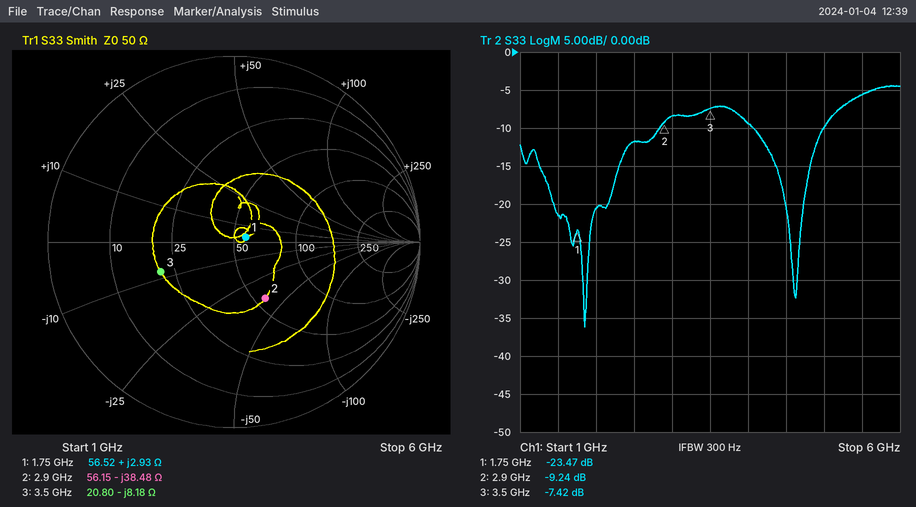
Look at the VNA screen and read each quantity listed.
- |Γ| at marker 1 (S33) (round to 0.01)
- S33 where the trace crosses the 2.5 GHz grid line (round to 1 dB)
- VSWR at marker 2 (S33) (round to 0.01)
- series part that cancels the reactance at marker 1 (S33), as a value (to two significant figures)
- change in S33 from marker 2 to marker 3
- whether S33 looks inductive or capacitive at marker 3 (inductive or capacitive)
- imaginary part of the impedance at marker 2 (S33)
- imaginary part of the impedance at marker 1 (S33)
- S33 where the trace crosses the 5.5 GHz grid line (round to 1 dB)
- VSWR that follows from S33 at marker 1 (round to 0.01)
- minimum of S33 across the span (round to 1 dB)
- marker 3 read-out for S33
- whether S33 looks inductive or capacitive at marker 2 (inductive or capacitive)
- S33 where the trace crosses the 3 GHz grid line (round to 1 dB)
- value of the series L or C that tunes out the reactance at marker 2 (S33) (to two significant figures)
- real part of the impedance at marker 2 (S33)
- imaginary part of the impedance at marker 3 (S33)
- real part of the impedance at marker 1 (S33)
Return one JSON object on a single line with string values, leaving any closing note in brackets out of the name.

{"|Γ| at marker 1 (S33)": "0.07", "S33 where the trace crosses the 2.5 GHz grid line": "-12 dB", "VSWR at marker 2 (S33)": "2.05", "series part that cancels the reactance at marker 1 (S33), as a value": "31 pF", "change in S33 from marker 2 to marker 3": "1.82 dB", "whether S33 looks inductive or capacitive at marker 3": "capacitive", "imaginary part of the impedance at marker 2": "-38.48 Ω", "imaginary part of the impedance at marker 1": "+2.93 Ω", "S33 where the trace crosses the 5.5 GHz grid line": "-6 dB", "VSWR that follows from S33 at marker 1": "1.14", "minimum of S33 across the span": "-36 dB", "marker 3 read-out for S33": "-7.42 dB", "whether S33 looks inductive or capacitive at marker 2": "capacitive", "S33 where the trace crosses the 3 GHz grid line": "-8 dB", "value of the series L or C that tunes out the reactance at marker 2 (S33)": "2.1 nH", "real part of the impedance at marker 2": "56.15 Ω", "imaginary part of the impedance at marker 3": "-8.18 Ω", "real part of the impedance at marker 1": "56.52 Ω"}
